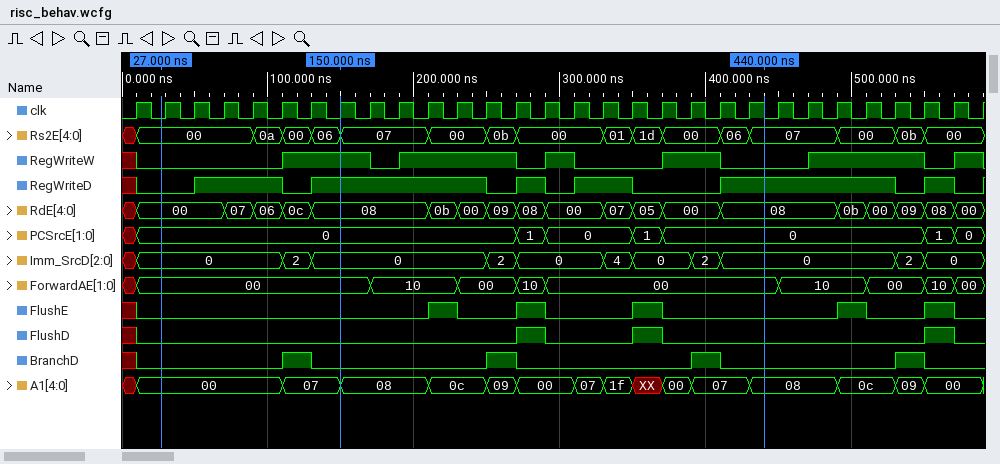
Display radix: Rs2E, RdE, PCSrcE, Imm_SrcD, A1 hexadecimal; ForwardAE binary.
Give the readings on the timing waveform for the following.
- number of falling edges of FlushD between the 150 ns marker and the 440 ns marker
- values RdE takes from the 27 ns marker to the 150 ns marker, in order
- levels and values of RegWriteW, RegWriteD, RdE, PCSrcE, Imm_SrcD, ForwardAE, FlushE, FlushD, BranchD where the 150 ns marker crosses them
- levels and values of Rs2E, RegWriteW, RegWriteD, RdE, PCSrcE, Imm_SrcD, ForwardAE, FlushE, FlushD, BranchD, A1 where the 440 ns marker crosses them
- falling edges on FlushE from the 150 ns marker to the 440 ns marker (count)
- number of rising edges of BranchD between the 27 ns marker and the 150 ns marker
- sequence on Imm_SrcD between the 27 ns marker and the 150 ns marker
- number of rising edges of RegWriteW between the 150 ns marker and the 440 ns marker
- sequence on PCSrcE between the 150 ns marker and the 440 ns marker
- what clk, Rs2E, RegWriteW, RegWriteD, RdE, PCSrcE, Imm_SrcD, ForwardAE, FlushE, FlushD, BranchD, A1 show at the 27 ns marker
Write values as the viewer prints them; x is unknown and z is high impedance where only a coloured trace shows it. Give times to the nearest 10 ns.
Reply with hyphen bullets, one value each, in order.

- 2
- 00, 07, 06, 0c, 08
- RegWriteW=1, RegWriteD=1, RdE=08, PCSrcE=0, Imm_SrcD=0, ForwardAE=00, FlushE=0, FlushD=0, BranchD=0
- Rs2E=07, RegWriteW=0, RegWriteD=1, RdE=08, PCSrcE=0, Imm_SrcD=0, ForwardAE=00, FlushE=0, FlushD=0, BranchD=0, A1=08
- 3
- 1
- 0, 2, 0
- 3
- 0, 1, 0, 1, 0
- clk=0, Rs2E=00, RegWriteW=0, RegWriteD=0, RdE=00, PCSrcE=0, Imm_SrcD=0, ForwardAE=00, FlushE=0, FlushD=0, BranchD=0, A1=00
